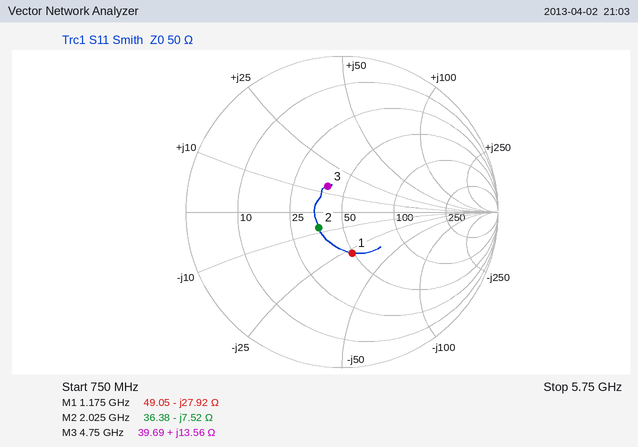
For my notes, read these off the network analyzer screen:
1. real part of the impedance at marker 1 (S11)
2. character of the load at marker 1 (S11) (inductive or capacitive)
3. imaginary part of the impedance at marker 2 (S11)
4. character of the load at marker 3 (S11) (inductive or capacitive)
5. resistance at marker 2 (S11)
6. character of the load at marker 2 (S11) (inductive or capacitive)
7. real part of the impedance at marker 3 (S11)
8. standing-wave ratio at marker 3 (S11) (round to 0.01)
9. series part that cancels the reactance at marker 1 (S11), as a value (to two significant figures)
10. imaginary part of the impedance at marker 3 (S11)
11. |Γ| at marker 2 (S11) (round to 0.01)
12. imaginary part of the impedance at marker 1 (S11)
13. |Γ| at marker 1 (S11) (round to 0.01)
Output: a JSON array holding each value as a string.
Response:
["49.05 Ω", "capacitive", "-7.52 Ω", "inductive", "36.38 Ω", "capacitive", "39.69 Ω", "1.46", "3.8 nH", "+13.56 Ω", "0.18", "-27.92 Ω", "0.27"]
